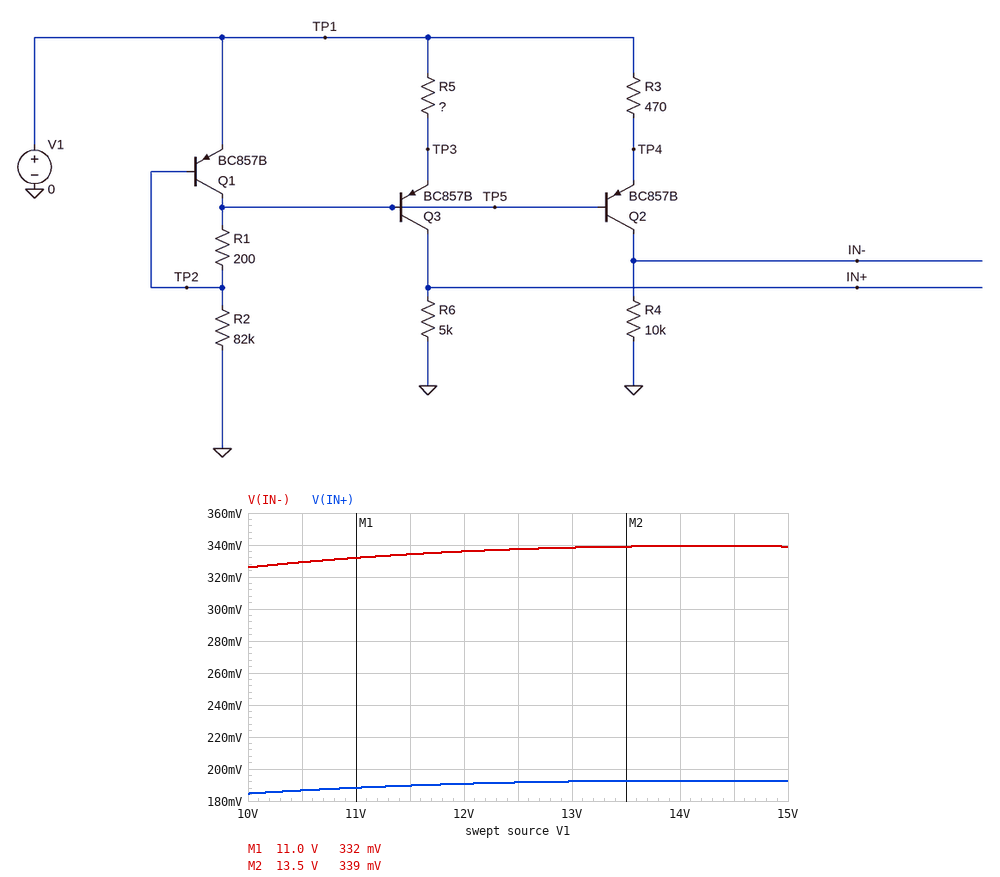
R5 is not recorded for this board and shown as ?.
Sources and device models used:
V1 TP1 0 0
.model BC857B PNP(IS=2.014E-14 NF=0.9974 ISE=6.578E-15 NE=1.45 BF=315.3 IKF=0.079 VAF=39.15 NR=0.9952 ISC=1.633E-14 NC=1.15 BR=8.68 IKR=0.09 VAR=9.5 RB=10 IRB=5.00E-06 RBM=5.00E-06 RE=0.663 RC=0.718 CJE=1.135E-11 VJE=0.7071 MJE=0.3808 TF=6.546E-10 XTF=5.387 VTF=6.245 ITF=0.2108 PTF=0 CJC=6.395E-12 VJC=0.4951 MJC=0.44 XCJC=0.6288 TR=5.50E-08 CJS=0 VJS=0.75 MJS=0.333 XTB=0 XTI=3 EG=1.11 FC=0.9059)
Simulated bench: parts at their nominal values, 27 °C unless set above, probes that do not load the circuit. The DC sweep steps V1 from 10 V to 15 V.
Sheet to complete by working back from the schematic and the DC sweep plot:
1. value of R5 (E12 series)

330 Ω
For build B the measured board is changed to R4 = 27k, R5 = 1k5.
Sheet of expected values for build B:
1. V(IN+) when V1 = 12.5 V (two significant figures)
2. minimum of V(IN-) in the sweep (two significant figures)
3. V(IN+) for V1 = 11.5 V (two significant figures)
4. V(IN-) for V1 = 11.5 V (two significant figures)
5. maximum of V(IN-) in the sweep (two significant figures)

99 mV
870 mV
98 mV
900 mV
910 mV
